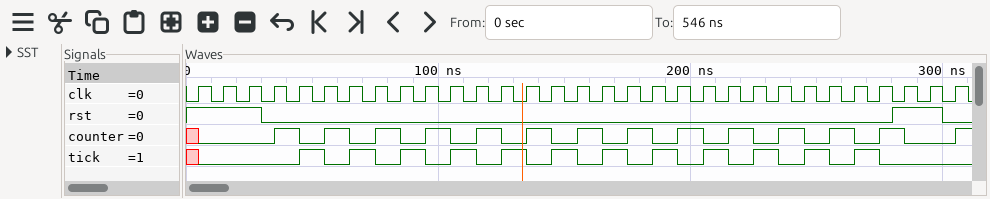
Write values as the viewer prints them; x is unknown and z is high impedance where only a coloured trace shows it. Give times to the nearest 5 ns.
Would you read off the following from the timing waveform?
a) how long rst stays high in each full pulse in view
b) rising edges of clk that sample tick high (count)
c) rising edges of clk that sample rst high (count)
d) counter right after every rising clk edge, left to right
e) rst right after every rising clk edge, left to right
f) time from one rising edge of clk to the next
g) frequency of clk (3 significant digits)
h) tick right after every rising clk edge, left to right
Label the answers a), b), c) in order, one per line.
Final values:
a) 20 ns
b) 12
c) 5
d) 0 0 0 1 0 1 0 1 0 1 0 1 0 1 0 1 0 1 0 1 0 1 0 1 0 1 0 1 0 0 1
e) 1 1 1 0 0 0 0 0 0 0 0 0 0 0 0 0 0 0 0 0 0 0 0 0 0 0 0 0 1 1 0
f) 10 ns
g) 100 MHz
h) 0 0 0 0 1 0 1 0 1 0 1 0 1 0 1 0 1 0 1 0 1 0 1 0 1 0 1 0 0 0 0
